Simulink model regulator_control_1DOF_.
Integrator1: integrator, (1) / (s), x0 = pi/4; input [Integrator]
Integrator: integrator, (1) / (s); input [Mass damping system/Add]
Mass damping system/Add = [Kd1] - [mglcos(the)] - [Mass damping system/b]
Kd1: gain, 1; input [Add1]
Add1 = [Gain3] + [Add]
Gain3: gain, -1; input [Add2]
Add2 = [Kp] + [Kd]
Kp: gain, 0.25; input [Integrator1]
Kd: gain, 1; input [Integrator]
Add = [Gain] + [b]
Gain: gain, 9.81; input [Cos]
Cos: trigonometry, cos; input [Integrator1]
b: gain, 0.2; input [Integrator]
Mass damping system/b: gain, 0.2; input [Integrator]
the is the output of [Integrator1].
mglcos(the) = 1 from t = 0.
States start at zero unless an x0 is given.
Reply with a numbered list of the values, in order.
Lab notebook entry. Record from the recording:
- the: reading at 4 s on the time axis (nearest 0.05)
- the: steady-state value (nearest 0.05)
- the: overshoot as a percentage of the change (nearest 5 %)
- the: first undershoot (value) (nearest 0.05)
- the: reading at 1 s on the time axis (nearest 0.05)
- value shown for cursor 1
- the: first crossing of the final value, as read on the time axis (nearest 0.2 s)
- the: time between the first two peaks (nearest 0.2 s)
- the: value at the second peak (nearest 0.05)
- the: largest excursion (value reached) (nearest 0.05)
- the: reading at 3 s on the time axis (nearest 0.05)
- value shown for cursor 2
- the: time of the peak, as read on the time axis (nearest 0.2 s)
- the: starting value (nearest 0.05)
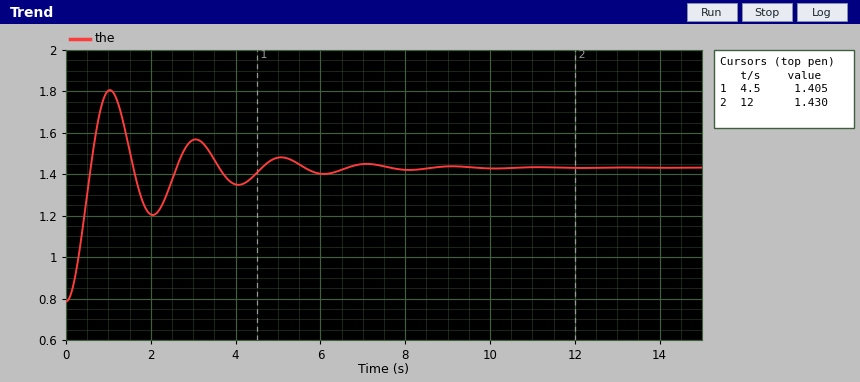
1. 1.35
2. 1.45
3. 60 %
4. 1.20
5. 1.80
6. 1.405
7. 0.6 s
8. 2.0 s
9. 1.55
10. 1.80
11. 1.55
12. 1.430
13. 1.0 s
14. 0.80
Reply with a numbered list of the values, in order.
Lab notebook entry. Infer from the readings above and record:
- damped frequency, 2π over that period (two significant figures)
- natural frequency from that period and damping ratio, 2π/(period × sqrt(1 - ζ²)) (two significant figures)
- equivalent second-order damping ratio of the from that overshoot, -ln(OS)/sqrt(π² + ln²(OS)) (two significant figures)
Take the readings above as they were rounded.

1. 3.1 rad/s
2. 3.2 rad/s
3. 0.16
